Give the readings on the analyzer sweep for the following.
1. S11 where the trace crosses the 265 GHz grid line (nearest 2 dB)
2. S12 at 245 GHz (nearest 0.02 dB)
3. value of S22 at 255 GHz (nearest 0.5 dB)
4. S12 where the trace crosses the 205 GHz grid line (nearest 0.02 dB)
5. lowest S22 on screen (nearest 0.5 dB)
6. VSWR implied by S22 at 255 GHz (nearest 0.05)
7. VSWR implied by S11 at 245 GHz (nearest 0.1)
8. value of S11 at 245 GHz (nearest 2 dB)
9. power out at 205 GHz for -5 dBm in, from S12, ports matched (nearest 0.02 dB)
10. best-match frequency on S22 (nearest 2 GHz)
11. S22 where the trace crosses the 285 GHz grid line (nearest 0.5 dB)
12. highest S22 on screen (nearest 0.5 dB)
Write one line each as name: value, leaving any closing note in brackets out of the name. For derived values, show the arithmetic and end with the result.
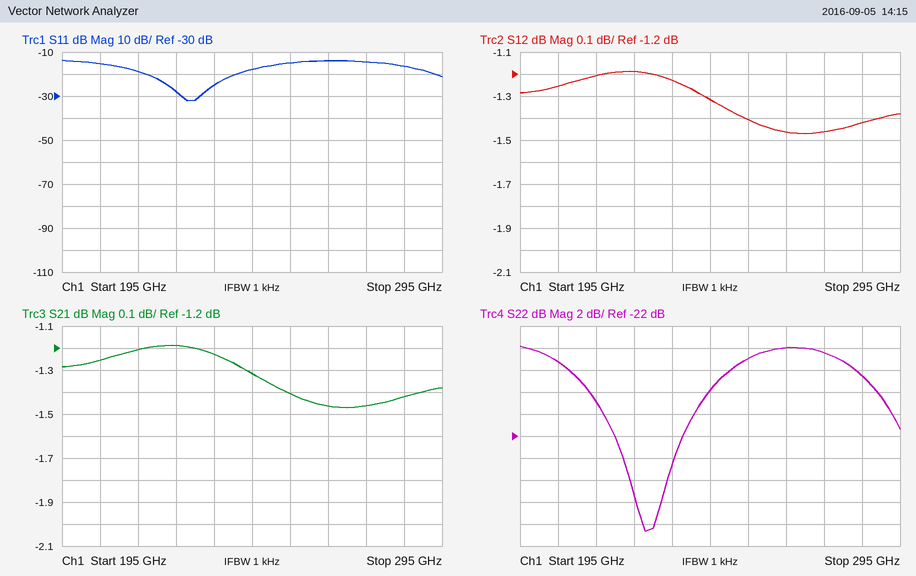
S11 where the trace crosses the 265 GHz grid line: -14 dB
S12 at 245 GHz: -1.32 dB
value of S22 at 255 GHz: -15.0 dB
S12 where the trace crosses the 205 GHz grid line: -1.26 dB
lowest S22 on screen: -30.5 dB
VSWR implied by S22 at 255 GHz: |Γ| = 10^(-15/20) = 0.1778; VSWR = (1 + 0.1778)/(1 − 0.1778) ≈ 1.43, so 1.45 to the nearest 0.05
VSWR implied by S11 at 245 GHz: |Γ| = 10^(-18/20) = 0.1259; VSWR = (1 + 0.1259)/(1 − 0.1259) ≈ 1.3
value of S11 at 245 GHz: -18 dB
power out at 205 GHz for -5 dBm in, from S12, ports matched: -5 dBm + (-1.26 dB) = -6.26 dBm
best-match frequency on S22: 228 GHz
S22 where the trace crosses the 285 GHz grid line: -16.5 dB
highest S22 on screen: -14.0 dB
